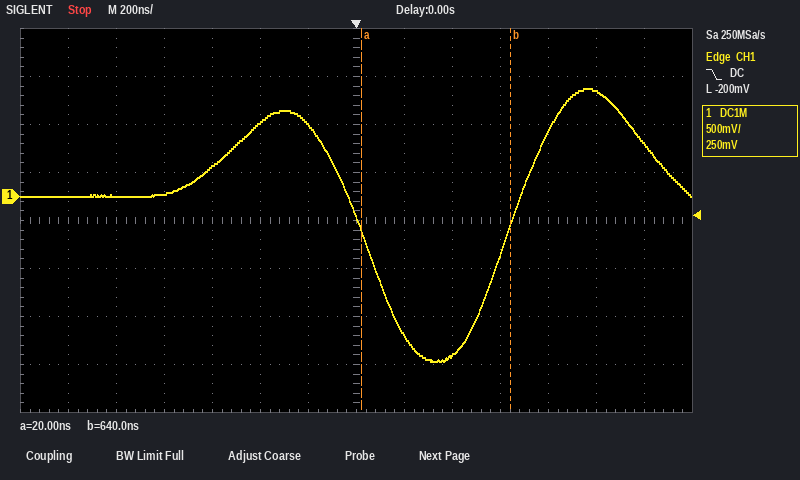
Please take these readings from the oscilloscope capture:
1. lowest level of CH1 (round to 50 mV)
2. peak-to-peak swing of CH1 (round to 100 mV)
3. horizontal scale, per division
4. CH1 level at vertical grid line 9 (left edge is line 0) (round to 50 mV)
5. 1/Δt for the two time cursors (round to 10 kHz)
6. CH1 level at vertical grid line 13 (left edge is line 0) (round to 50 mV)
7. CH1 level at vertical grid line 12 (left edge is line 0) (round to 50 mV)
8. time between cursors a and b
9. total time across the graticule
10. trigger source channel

-1.70 V
2.80 V
200 ns
-1.65 V
1.61 MHz
550 mV
1.10 V
620 ns
2.8 µs
CH1
